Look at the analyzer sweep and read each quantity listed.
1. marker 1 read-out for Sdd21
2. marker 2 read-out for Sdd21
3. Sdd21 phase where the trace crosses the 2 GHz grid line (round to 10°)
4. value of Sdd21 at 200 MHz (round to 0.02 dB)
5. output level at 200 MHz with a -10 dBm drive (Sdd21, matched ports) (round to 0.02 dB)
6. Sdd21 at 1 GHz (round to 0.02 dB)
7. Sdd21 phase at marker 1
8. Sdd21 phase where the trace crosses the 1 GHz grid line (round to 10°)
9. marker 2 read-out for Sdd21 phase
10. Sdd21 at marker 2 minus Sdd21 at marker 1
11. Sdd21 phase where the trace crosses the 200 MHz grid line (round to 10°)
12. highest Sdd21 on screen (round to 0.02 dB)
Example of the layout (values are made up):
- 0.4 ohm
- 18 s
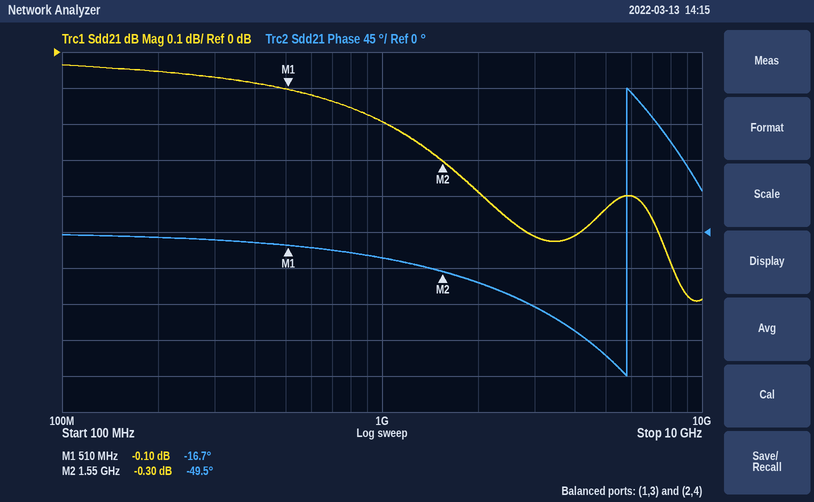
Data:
- -0.10 dB
- -0.30 dB
- -60°
- -0.06 dB
- -10.06 dBm
- -0.20 dB
- -16.7°
- -30°
- -49.5°
- -0.20 dB
- -10°
- -0.04 dB
